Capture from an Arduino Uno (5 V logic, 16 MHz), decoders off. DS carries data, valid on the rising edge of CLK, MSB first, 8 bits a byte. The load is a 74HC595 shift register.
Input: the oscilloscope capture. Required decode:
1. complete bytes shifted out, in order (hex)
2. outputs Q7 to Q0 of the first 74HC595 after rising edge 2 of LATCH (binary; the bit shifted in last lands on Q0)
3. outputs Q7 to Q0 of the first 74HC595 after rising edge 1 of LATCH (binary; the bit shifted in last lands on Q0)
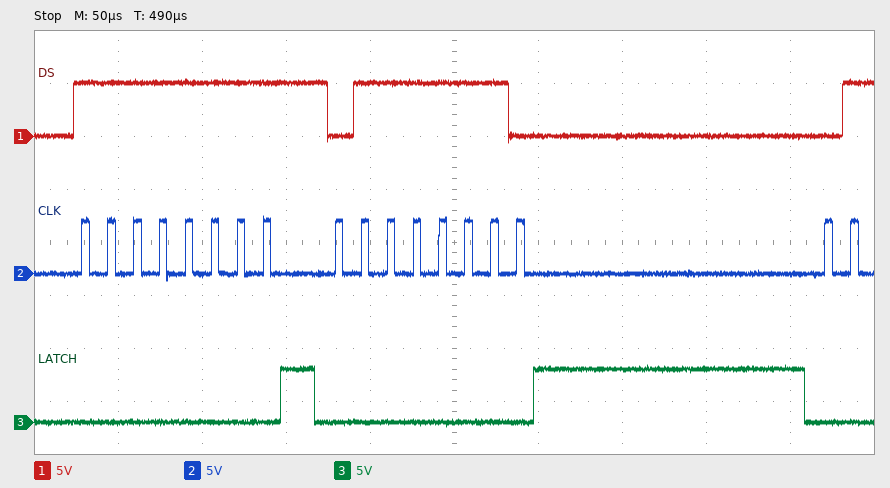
0xFF 0x7E
01111110
11111111
